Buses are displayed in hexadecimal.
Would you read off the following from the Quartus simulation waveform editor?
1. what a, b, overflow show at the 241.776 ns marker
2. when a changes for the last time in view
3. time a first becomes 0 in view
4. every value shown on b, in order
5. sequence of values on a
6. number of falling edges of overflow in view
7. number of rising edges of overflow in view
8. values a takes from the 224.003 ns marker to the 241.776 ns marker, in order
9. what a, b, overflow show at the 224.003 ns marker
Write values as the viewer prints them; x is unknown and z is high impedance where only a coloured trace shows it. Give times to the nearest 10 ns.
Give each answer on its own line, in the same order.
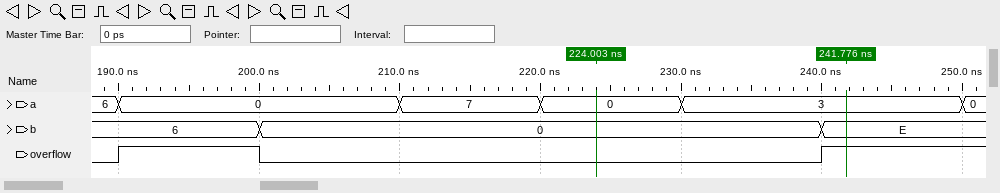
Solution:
a=3, b=E, overflow=1
250 ns
190 ns
6, 0, E
6, 0, 7, 0, 3, 0
1
2
0, 3
a=0, b=0, overflow=0
